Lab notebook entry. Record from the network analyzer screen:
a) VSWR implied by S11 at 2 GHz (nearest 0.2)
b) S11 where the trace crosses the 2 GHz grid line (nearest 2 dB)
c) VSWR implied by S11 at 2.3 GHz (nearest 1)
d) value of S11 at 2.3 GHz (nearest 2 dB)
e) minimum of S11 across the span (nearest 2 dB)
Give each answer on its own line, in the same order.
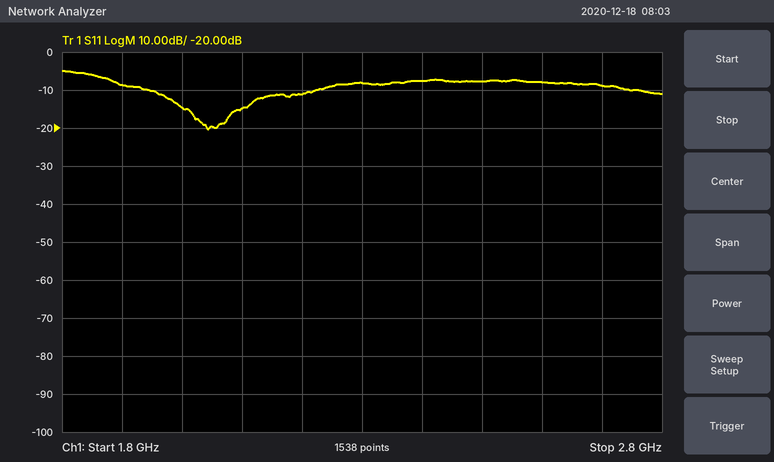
1.4
-14 dB
2
-8 dB
-20 dB
